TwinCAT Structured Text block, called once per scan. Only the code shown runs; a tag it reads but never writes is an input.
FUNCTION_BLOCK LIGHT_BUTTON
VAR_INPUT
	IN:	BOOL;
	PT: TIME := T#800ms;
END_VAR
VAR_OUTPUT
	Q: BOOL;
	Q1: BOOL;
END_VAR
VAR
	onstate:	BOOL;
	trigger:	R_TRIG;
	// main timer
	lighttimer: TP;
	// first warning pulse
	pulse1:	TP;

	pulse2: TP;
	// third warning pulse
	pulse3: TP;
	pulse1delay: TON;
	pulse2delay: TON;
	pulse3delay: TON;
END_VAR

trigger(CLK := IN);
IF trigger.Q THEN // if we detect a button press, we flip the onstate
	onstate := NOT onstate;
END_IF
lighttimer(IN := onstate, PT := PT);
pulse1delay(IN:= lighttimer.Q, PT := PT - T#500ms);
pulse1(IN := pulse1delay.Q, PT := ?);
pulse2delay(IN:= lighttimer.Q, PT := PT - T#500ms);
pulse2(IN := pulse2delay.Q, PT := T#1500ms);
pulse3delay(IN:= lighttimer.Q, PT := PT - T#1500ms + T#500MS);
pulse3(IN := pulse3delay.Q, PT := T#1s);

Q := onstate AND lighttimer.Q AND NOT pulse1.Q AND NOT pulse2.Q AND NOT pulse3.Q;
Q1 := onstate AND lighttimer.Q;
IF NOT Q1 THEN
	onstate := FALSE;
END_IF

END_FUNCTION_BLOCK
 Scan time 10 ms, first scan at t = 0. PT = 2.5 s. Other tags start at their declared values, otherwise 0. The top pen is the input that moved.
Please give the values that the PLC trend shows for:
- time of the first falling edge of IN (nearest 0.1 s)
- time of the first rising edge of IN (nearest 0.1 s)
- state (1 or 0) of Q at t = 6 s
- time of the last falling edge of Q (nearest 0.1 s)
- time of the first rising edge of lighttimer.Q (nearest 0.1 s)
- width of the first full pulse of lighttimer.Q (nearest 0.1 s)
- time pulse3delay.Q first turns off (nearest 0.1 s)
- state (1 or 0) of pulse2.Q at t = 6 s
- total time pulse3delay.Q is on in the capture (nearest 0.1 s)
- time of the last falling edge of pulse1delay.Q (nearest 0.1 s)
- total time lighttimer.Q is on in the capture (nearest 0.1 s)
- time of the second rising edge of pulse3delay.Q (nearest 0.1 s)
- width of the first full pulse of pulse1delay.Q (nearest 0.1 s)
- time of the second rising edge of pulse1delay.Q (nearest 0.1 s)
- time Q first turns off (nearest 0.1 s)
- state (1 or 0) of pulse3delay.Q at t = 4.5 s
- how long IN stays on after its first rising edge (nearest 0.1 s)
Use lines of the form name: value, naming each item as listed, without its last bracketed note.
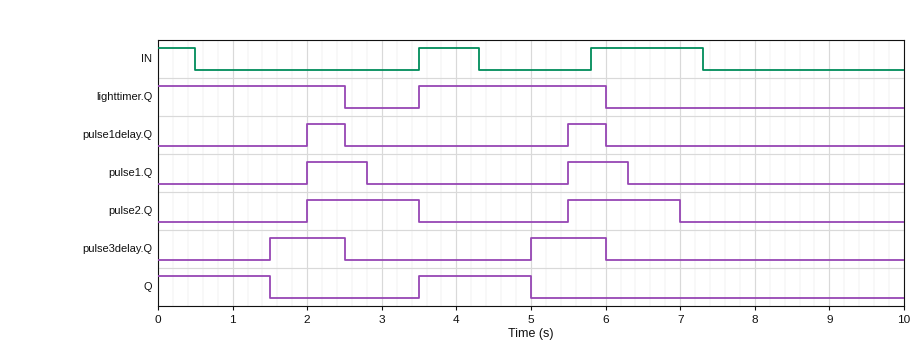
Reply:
time of the first falling edge of IN: 0.5 s
time of the first rising edge of IN: 3.5 s
state (1 or 0) of Q at t = 6 s: 0
time of the last falling edge of Q: 5.0 s
time of the first rising edge of lighttimer.Q: 3.5 s
width of the first full pulse of lighttimer.Q: 2.5 s
time pulse3delay.Q first turns off: 2.5 s
state (1 or 0) of pulse2.Q at t = 6 s: 1
total time pulse3delay.Q is on in the capture: 2.0 s
time of the last falling edge of pulse1delay.Q: 6.0 s
total time lighttimer.Q is on in the capture: 5.0 s
time of the second rising edge of pulse3delay.Q: 5.0 s
width of the first full pulse of pulse1delay.Q: 0.5 s
time of the second rising edge of pulse1delay.Q: 5.5 s
time Q first turns off: 1.5 s
state (1 or 0) of pulse3delay.Q at t = 4.5 s: 0
how long IN stays on after its first rising edge: 0.8 s
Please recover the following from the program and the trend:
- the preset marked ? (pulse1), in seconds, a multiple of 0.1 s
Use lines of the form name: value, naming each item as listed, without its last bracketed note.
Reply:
the preset marked ? (pulse1), in seconds, a multiple of 0.1 s: 0.8 s
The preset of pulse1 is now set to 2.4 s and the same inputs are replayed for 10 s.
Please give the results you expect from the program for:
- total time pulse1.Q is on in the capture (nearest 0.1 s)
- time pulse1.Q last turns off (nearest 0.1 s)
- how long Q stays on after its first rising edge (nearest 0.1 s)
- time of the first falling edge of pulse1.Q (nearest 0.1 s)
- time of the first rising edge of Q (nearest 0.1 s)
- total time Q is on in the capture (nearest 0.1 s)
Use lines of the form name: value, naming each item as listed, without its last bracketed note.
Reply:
total time pulse1.Q is on in the capture: 4.8 s
time pulse1.Q last turns off: 7.9 s
how long Q stays on after its first rising edge: 0.6 s
time of the first falling edge of pulse1.Q: 4.4 s
time of the first rising edge of Q: 4.4 s
total time Q is on in the capture: 2.1 s
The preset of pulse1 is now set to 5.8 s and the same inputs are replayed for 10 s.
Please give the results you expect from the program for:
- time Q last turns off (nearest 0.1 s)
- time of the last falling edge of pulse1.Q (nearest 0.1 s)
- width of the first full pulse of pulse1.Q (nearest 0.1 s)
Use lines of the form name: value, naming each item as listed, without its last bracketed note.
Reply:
time Q last turns off: 1.5 s
time of the last falling edge of pulse1.Q: 7.8 s
width of the first full pulse of pulse1.Q: 5.8 s
